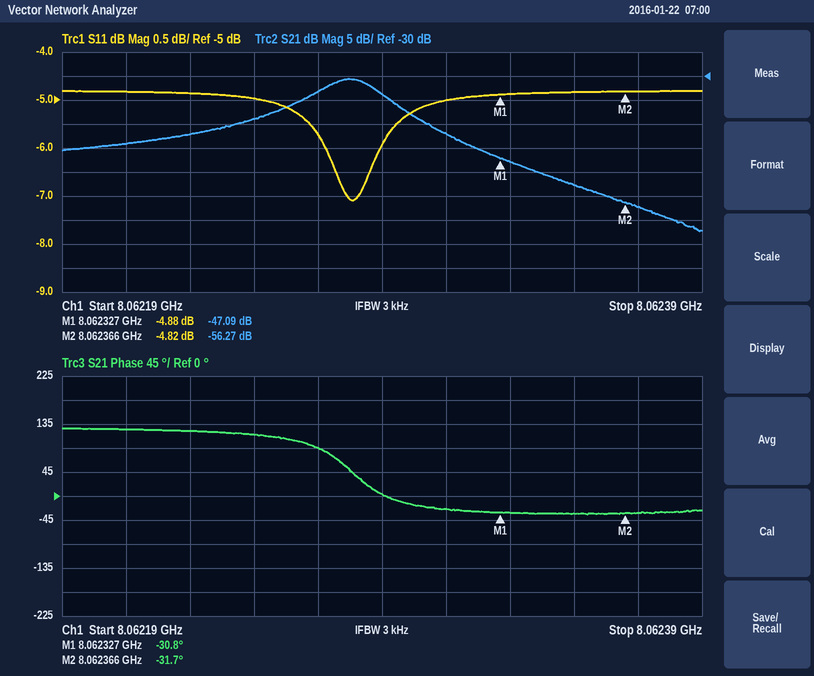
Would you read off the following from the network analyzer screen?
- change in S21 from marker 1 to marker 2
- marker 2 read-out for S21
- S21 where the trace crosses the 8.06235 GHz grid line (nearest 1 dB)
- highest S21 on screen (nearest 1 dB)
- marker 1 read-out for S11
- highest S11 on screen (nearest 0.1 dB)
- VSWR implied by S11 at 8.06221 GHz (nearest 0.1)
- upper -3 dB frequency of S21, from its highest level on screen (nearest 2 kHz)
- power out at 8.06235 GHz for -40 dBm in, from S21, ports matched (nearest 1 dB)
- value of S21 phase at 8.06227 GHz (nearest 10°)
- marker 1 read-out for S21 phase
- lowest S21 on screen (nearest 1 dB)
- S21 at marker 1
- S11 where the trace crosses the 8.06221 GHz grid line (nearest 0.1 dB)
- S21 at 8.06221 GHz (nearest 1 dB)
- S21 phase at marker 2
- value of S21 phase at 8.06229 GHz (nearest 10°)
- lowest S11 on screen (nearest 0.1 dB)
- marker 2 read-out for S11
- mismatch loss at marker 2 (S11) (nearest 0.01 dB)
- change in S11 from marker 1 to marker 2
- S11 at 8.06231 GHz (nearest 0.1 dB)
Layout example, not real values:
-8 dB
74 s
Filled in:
-9.18 dB
-56.27 dB
-53 dB
-31 dB
-4.88 dB
-4.8 dB
3.7
8.062290 GHz
-93 dBm
90°
-30.8°
-62 dB
-47.09 dB
-4.8 dB
-44 dB
-31.7°
0°
-7.1 dB
-4.82 dB
1.74 dB
0.06 dB
-5.0 dB
